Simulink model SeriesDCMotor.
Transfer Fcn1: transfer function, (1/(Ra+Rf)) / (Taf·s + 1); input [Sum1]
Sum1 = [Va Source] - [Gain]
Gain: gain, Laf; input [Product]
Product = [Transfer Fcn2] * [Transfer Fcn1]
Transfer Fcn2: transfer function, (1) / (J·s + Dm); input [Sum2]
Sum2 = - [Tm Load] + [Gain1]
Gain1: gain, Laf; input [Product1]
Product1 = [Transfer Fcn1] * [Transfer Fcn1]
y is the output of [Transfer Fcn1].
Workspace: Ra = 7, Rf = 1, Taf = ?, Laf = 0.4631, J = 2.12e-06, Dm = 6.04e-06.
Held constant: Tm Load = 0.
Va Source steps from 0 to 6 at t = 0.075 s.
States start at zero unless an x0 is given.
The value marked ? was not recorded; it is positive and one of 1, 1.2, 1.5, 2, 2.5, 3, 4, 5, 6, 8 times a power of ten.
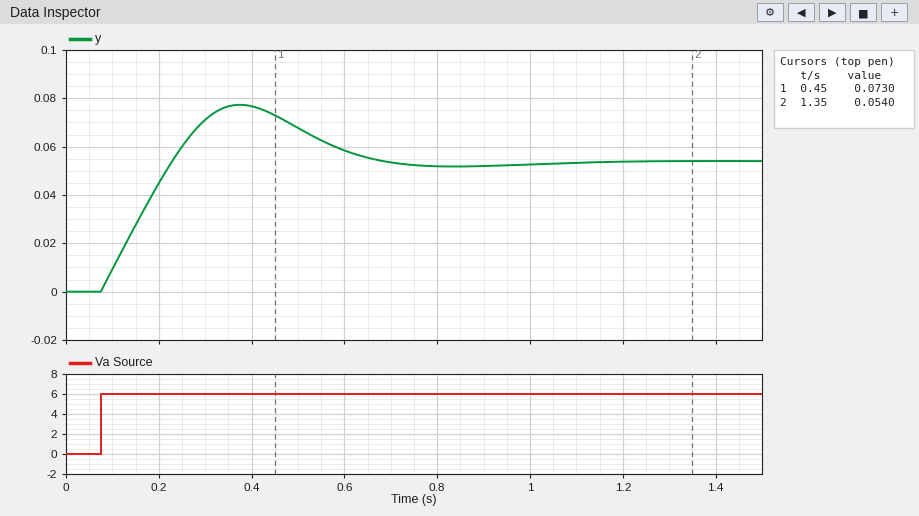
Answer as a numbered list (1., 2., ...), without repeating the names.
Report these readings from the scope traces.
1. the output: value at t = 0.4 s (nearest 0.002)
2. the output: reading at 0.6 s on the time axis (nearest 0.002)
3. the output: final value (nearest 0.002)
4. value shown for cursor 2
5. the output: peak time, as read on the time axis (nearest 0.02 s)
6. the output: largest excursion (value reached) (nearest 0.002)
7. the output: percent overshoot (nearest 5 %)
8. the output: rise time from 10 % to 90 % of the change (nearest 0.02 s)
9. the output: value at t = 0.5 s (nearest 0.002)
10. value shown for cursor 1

1. 0.076
2. 0.058
3. 0.054
4. 0.0540
5. 0.38 s
6. 0.078
7. 45 %
8. 0.12 s
9. 0.068
10. 0.0730
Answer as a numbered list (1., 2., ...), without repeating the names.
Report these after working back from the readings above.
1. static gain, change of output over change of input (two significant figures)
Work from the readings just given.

1. 0.0090
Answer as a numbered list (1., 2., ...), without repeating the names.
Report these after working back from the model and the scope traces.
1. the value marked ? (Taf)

1. 2
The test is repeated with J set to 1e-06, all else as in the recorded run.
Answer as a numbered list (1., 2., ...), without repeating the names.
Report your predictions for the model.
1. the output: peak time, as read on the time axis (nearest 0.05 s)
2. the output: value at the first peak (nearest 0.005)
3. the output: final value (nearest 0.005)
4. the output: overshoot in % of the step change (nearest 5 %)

1. 0.35 s
2. 0.065
3. 0.055
4. 25 %
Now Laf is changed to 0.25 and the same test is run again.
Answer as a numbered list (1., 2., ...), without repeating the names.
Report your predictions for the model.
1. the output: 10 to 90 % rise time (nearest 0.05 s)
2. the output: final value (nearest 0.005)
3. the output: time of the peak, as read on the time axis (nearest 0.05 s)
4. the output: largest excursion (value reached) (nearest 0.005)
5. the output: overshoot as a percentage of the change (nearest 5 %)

1. 0.20 s
2. 0.080
3. 0.50 s
4. 0.105
5. 30 %
